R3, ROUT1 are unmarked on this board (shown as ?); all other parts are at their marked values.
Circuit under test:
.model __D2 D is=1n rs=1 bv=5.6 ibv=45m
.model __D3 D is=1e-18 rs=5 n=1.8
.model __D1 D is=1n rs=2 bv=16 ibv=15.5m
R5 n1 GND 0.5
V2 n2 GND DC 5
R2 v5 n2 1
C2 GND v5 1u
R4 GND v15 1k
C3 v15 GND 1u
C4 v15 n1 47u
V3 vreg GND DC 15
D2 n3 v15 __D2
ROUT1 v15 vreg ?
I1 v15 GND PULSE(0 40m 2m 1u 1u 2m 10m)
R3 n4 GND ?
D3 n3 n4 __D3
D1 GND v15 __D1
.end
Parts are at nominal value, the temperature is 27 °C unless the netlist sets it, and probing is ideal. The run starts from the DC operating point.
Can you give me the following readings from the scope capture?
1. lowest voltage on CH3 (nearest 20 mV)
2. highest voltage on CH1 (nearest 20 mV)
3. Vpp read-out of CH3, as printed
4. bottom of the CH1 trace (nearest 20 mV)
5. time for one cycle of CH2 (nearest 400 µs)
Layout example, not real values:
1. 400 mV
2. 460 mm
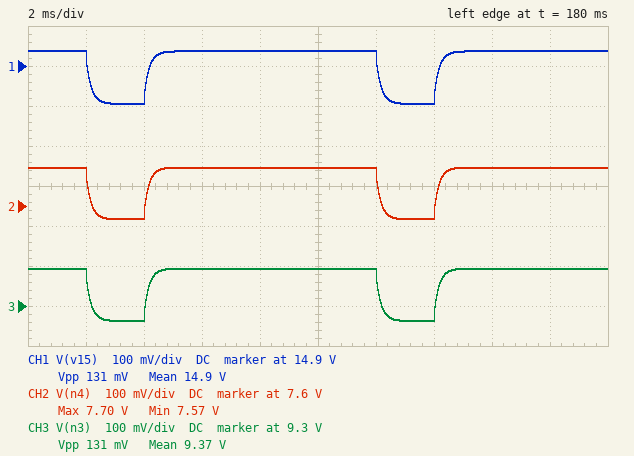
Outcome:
1. 9.26 V
2. 14.94 V
3. 131 mV
4. 14.80 V
5. 10.0 ms
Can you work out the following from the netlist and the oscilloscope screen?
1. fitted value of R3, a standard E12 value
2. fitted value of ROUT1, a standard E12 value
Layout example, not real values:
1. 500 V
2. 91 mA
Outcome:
1. 1.8 kΩ
2. 3.3 Ω
